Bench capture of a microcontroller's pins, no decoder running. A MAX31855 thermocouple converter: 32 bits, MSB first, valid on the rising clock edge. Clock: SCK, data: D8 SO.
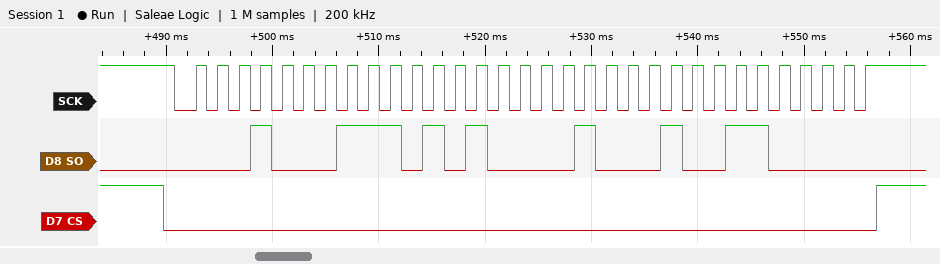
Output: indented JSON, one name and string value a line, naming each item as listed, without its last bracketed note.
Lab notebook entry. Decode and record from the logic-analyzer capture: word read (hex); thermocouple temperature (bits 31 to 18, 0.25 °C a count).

{
  "word read": "0x11D42260",
  "thermocouple temperature": "285.25 °C"
}
